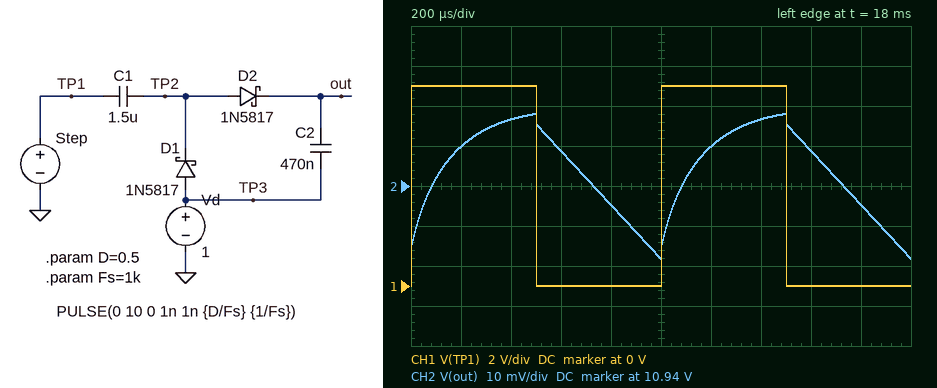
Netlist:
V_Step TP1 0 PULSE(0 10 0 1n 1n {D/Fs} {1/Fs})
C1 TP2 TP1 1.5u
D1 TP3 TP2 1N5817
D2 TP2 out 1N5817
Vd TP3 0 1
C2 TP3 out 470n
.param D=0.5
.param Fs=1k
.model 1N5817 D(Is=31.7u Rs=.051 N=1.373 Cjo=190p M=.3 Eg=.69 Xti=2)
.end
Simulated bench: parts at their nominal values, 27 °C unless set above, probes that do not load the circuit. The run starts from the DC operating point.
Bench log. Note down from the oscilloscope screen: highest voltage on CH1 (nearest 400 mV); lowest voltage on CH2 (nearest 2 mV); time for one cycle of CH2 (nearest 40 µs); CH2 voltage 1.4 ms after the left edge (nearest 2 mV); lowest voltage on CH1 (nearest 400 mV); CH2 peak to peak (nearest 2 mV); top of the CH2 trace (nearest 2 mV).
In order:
10.0 V
10.922 V
1.00 ms
10.956 V
0 V
36 mV
10.958 V
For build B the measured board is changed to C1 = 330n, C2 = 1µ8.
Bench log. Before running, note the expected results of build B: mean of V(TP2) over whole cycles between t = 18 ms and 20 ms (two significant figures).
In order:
5.8 V
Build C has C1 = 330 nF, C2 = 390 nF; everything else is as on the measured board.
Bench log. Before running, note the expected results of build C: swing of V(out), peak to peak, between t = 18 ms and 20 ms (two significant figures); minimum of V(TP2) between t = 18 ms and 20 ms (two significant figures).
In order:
48 mV
920 mV
